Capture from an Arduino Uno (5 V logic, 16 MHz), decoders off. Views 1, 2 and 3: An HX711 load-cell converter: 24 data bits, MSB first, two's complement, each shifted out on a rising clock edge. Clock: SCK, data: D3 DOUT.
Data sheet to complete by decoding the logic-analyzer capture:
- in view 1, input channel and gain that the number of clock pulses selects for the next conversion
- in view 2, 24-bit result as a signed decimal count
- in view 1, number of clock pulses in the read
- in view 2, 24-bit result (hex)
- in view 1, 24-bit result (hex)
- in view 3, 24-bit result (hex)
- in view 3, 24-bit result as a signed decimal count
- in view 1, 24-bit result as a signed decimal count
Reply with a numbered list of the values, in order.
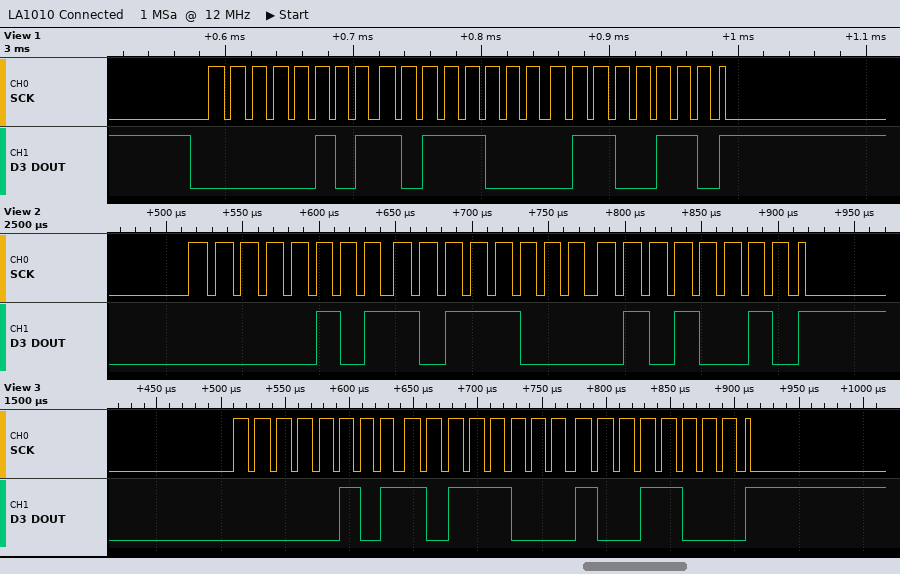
1. channel A, gain 128
2. 374866
3. 25
4. 0x05B852
5. 0x05B866
6. 0x05B898
7. 374936
8. 374886
